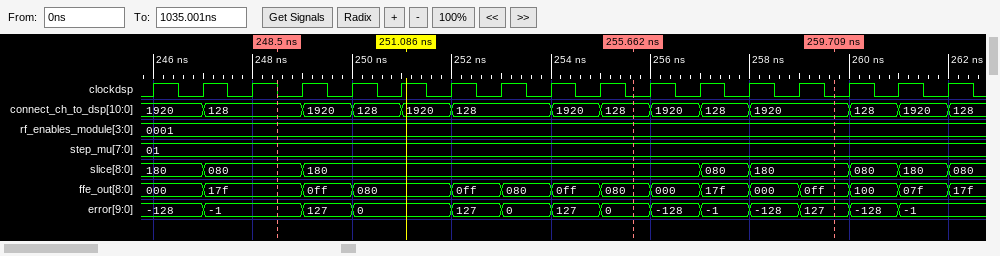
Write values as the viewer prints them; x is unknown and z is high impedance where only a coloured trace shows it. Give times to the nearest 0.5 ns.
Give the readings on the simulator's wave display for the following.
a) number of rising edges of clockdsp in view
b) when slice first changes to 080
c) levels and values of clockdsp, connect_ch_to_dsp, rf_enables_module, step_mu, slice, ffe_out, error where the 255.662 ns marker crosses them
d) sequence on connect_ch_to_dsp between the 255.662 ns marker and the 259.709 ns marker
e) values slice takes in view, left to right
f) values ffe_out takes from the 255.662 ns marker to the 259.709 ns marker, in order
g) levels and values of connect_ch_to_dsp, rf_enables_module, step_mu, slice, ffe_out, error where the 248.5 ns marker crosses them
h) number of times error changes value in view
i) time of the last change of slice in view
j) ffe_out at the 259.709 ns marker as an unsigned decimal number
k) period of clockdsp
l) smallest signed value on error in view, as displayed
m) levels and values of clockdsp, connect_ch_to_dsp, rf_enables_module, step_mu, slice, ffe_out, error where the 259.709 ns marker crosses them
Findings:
17
247 ns
clockdsp=0, connect_ch_to_dsp=128, rf_enables_module=0001, step_mu=01, slice=180, ffe_out=080, error=0
128, 1920, 128, 1920
180, 080, 180, 080, 180, 080, 180, 080
080, 000, 17f, 000, 0ff
connect_ch_to_dsp=128, rf_enables_module=0001, step_mu=01, slice=080, ffe_out=17f, error=-1
13
262 ns
255
1 ns
-128
clockdsp=0, connect_ch_to_dsp=1920, rf_enables_module=0001, step_mu=01, slice=180, ffe_out=0ff, error=127
